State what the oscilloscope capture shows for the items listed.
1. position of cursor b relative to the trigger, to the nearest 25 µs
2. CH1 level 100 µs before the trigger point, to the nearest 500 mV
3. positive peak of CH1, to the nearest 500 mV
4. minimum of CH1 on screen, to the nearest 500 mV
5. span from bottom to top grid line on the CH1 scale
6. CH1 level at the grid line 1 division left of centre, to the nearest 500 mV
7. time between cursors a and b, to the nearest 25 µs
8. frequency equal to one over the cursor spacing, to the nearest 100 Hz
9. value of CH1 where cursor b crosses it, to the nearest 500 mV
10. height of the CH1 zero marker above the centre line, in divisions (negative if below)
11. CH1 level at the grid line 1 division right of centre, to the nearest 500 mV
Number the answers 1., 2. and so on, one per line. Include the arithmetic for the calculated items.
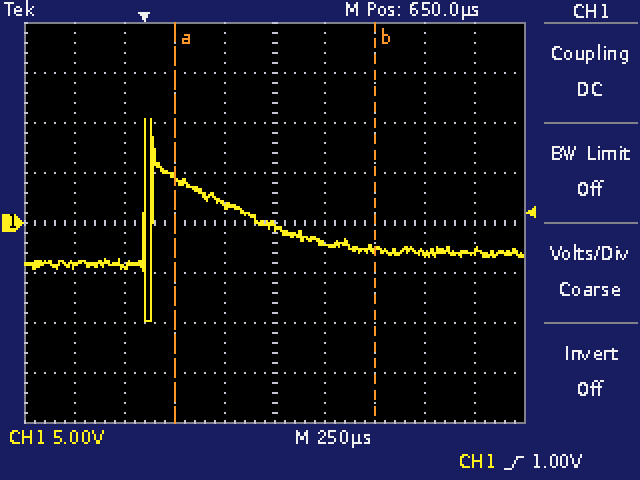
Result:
1. +1.150 ms
2. -4.5 V
3. 10.5 V
4. -10.0 V
5. 40 V
6. 2.0 V
7. 1.000 ms
8. 1 / 1.000 ms ≈ 1.0 kHz
9. -2.5 V
10. 0.0 div
11. -2.0 V
